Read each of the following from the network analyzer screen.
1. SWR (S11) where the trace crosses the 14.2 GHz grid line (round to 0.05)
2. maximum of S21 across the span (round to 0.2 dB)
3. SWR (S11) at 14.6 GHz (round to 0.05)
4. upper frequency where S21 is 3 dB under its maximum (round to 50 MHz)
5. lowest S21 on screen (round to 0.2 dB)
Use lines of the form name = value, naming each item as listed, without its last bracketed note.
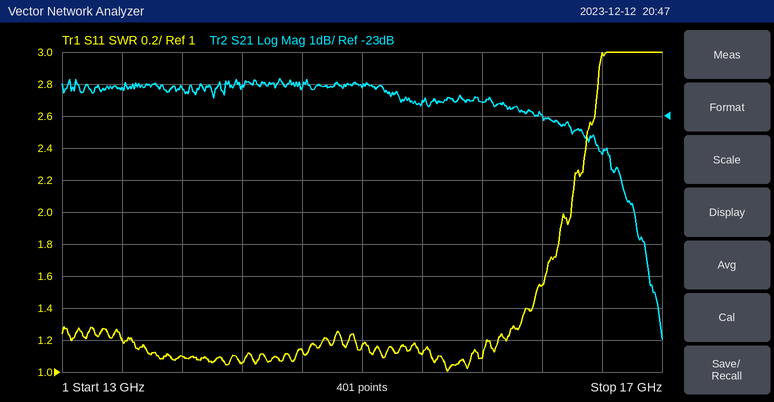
SWR (S11) where the trace crosses the 14.2 GHz grid line = 1.05
maximum of S21 across the span = -21.8 dB
SWR (S11) at 14.6 GHz = 1.15
upper frequency where S21 is 3 dB under its maximum = 16.70 GHz
lowest S21 on screen = -30.0 dB
